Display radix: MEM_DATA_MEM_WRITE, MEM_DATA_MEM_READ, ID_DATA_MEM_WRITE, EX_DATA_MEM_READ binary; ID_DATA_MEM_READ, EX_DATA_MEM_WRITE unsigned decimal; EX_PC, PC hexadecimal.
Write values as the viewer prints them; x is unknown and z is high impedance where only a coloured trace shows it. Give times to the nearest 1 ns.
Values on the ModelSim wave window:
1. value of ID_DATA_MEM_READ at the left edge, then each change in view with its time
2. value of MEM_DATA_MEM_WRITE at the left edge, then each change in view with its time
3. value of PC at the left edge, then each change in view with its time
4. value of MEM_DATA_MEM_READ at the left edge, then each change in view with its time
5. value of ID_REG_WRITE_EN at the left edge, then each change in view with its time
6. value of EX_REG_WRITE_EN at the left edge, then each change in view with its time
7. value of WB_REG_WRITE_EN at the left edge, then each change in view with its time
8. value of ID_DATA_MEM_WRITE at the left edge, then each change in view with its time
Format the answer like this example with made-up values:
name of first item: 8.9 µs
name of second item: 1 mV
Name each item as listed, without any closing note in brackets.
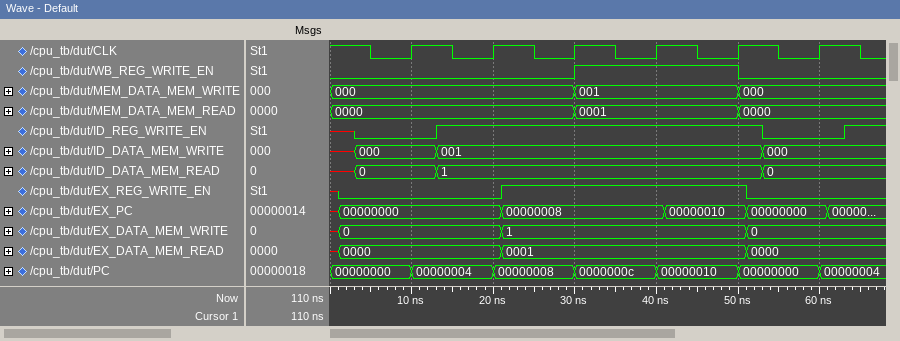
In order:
value of ID_DATA_MEM_READ at the left edge, then each change in view with its time: x, 0 at 3 ns, 1 at 13 ns, 0 at 53 ns
value of MEM_DATA_MEM_WRITE at the left edge, then each change in view with its time: 000, 001 at 30 ns, 000 at 50 ns
value of PC at the left edge, then each change in view with its time: 00000000, 00000004 at 10 ns, 00000008 at 20 ns, 0000000c at 30 ns, 00000010 at 40 ns, 00000000 at 50 ns, 00000004 at 60 ns
value of MEM_DATA_MEM_READ at the left edge, then each change in view with its time: 0000, 0001 at 30 ns, 0000 at 50 ns
value of ID_REG_WRITE_EN at the left edge, then each change in view with its time: x, 0 at 3 ns, 1 at 13 ns, 0 at 53 ns, 1 at 63 ns
value of EX_REG_WRITE_EN at the left edge, then each change in view with its time: x, 0 at 1 ns, 1 at 21 ns, 0 at 51 ns
value of WB_REG_WRITE_EN at the left edge, then each change in view with its time: 0, 1 at 30 ns, 0 at 50 ns
value of ID_DATA_MEM_WRITE at the left edge, then each change in view with its time: x, 000 at 3 ns, 001 at 13 ns, 000 at 53 ns
